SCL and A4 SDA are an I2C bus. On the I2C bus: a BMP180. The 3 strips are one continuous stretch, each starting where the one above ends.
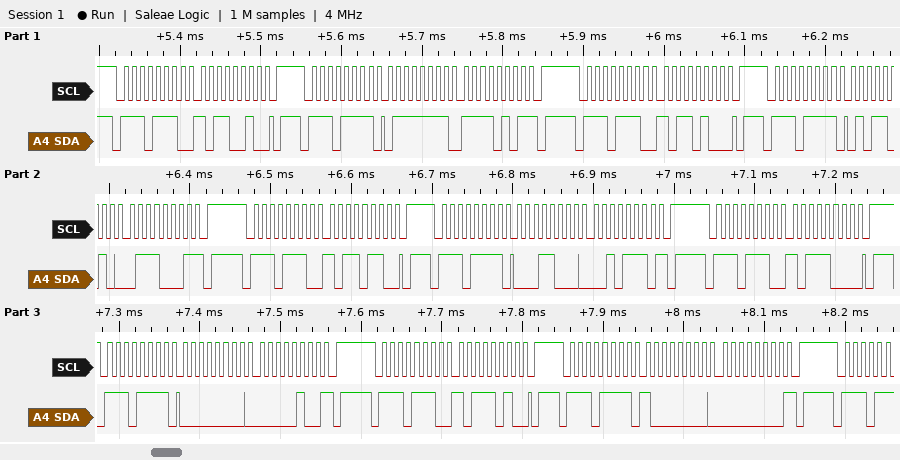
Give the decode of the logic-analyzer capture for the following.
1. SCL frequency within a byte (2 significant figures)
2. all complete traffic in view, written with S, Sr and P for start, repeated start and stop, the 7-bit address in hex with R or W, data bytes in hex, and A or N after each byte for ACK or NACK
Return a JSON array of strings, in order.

["100 kHz", "S 77W A B2 A P S 77R A 7F A F5 N P S 77W A B4 A P S 77R A 5A A 71 N P S 77W A B6 A P S 77R A 18 A 2E N P S 77W A B8 A P S 77R A 00 A 04 N P S 77W A BA A P S 77R A 80 A 00 N P"]
